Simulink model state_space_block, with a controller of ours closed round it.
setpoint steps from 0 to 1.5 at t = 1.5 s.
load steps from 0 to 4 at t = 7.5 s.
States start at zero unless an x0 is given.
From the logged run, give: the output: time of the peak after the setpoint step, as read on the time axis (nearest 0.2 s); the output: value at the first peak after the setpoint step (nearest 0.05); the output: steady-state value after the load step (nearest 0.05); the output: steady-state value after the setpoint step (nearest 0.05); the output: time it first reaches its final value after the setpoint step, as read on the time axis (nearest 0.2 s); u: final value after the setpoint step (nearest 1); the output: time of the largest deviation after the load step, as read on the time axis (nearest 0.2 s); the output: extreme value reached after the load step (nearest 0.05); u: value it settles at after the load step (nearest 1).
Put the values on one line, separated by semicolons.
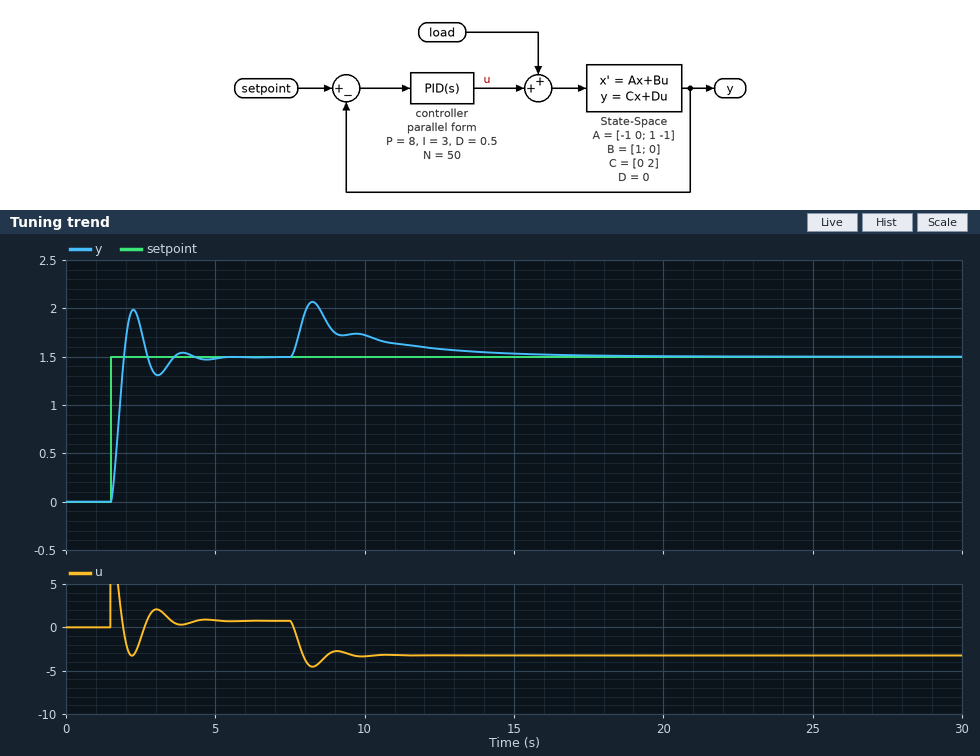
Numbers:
2.2 s; 2.00; 1.50; 1.50; 2.0 s; 1; 8.2 s; 2.05; -3
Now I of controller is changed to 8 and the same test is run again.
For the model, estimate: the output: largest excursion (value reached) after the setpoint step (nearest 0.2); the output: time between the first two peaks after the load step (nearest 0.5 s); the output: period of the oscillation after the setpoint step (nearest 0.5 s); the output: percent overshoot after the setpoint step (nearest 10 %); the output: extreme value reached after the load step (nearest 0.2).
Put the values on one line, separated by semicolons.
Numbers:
2.2; 1.5 s; 1.5 s; 50 %; 2.0
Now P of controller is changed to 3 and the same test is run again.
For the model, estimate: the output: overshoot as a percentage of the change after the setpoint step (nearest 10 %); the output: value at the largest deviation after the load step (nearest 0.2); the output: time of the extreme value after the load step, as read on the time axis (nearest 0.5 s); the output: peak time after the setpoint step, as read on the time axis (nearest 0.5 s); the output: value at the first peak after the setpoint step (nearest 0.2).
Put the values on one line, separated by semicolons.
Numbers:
30 %; 2.6; 8.5 s; 3.0 s; 2.0
